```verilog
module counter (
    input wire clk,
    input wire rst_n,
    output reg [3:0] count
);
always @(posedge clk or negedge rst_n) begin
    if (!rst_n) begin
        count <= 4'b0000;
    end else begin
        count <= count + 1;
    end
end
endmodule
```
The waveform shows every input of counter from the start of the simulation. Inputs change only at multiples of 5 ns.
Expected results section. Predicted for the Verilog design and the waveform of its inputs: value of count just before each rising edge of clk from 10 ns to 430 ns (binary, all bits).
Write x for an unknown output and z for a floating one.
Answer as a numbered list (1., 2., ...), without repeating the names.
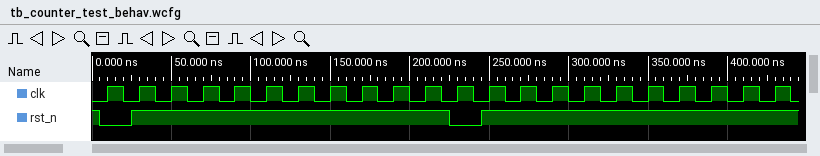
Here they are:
1. 0000, 0000, 0001, 0010, 0011, 0100, 0101, 0110, 0111, 1000, 1001, 0000, 0000, 0001, 0010, 0011, 0100, 0101, 0110, 0111, 1000, 1001
